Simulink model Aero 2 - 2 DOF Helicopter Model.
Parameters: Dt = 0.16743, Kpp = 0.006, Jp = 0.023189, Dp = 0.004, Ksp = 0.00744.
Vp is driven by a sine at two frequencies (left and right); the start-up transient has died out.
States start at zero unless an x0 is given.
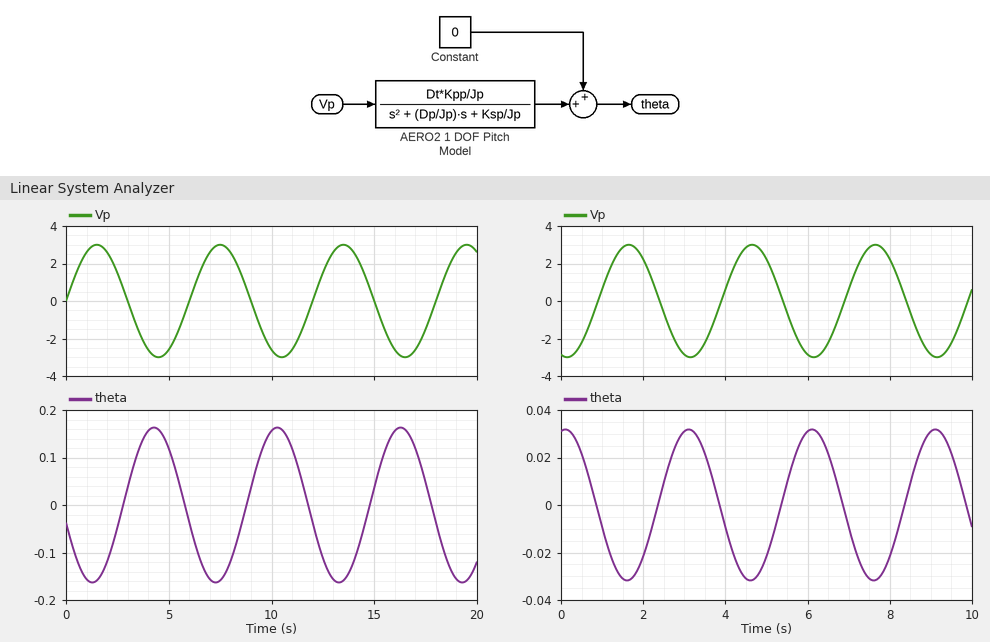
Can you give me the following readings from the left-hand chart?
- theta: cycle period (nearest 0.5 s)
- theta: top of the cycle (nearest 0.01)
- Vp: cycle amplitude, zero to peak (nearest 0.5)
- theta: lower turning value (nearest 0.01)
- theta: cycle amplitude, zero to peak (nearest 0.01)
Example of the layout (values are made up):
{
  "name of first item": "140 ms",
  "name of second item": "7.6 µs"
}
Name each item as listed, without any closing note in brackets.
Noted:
{
  "theta: cycle period": "6.0 s",
  "theta: top of the cycle": "0.16",
  "Vp: cycle amplitude, zero to peak": "3.0",
  "theta: lower turning value": "-0.16",
  "theta: cycle amplitude, zero to peak": "0.16"
}
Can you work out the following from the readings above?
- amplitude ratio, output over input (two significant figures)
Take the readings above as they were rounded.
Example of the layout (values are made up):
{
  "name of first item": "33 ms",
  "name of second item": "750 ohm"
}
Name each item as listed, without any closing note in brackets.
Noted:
{
  "amplitude ratio, output over input": "0.053"
}
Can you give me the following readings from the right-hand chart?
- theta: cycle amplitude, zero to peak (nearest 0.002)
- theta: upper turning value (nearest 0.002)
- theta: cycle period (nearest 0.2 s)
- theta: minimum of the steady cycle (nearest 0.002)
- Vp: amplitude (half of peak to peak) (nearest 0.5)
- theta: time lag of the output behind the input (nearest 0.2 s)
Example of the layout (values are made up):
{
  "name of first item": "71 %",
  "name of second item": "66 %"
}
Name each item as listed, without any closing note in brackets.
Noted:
{
  "theta: cycle amplitude, zero to peak": "0.032",
  "theta: upper turning value": "0.032",
  "theta: cycle period": "3.0 s",
  "theta: minimum of the steady cycle": "-0.032",
  "Vp: amplitude (half of peak to peak)": "3.0",
  "theta: time lag of the output behind the input": "1.4 s"
}
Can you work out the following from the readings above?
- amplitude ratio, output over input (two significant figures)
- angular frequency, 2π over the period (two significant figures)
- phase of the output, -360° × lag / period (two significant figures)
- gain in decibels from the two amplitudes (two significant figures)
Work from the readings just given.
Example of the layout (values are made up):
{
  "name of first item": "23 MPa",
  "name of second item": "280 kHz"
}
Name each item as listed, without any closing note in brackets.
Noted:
{
  "amplitude ratio, output over input": "0.011",
  "angular frequency, 2π over the period": "2.1 rad/s",
  "phase of the output, -360° × lag / period": "-170°",
  "gain in decibels from the two amplitudes": "-39 dB"
}
